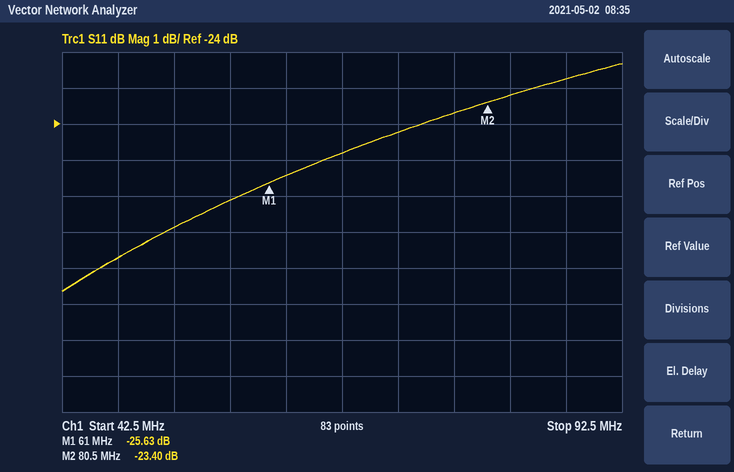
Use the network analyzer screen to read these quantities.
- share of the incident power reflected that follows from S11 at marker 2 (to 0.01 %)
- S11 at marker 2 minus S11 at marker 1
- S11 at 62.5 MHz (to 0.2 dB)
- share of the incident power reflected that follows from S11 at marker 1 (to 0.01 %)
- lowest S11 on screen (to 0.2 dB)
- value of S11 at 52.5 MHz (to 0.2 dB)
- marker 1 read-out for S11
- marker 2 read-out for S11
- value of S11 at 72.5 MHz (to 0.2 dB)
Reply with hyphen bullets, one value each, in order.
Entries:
- 0.46 %
- 2.23 dB
- -25.4 dB
- 0.27 %
- -28.6 dB
- -26.8 dB
- -25.63 dB
- -23.40 dB
- -24.2 dB
